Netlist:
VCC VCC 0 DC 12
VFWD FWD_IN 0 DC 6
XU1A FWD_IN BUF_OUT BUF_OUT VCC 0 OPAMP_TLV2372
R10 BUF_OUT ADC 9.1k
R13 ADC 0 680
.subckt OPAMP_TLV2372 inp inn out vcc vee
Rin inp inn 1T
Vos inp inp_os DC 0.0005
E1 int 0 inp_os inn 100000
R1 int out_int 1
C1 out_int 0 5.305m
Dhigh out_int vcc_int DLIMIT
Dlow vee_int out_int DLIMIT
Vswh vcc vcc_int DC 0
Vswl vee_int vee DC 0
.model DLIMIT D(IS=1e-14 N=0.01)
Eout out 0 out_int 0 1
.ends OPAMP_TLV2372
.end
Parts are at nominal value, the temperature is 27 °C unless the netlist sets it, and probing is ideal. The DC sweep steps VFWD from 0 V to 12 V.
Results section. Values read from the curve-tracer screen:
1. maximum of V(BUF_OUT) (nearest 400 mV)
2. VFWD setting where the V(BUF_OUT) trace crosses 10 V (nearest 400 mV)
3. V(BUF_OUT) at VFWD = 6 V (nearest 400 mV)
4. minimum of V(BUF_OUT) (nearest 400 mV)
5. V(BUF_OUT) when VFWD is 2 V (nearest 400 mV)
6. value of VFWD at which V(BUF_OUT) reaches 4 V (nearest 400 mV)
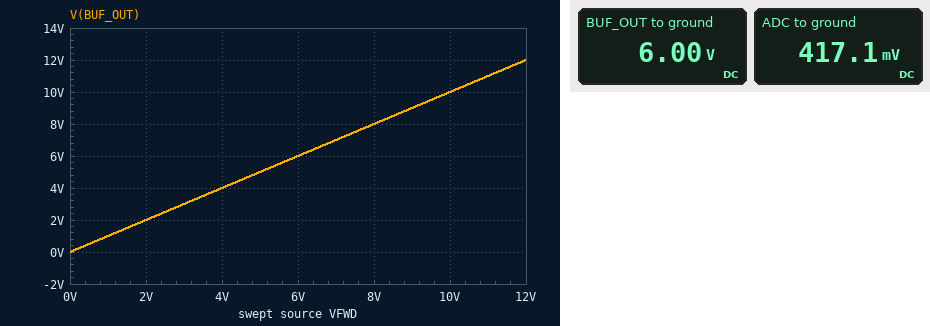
12.0 V
10.0 V
6.0 V
0 V
2.0 V
4.0 V
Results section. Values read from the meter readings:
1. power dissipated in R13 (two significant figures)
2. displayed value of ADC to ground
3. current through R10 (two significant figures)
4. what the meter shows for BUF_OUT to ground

260 µW
417.1 mV
610 µA
6.00 V
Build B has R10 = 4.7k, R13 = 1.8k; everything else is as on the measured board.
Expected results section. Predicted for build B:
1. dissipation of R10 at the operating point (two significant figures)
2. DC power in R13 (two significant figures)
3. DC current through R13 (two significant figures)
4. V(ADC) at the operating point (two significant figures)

4.0 mW
1.5 mW
920 µA
1.7 V
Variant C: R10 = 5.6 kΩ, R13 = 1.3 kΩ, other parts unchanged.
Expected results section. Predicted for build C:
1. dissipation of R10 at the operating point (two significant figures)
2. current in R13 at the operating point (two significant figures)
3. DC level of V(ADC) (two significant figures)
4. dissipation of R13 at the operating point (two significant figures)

4.2 mW
870 µA
1.1 V
980 µW
